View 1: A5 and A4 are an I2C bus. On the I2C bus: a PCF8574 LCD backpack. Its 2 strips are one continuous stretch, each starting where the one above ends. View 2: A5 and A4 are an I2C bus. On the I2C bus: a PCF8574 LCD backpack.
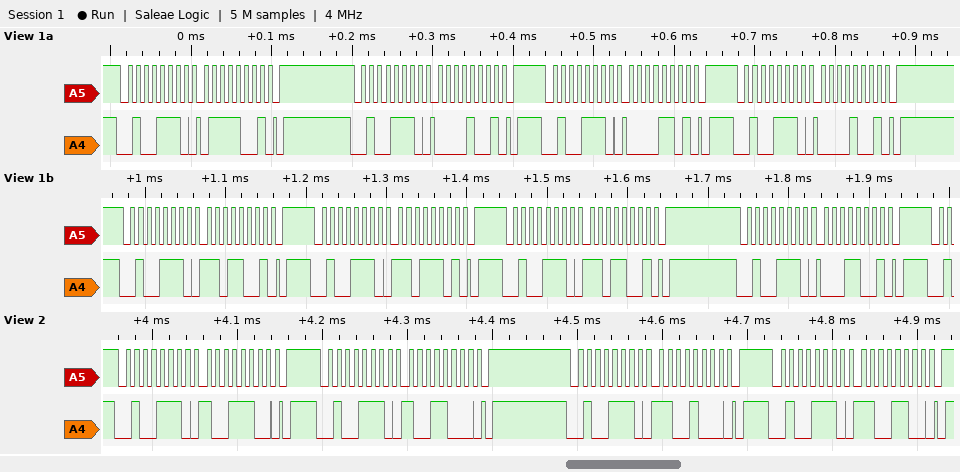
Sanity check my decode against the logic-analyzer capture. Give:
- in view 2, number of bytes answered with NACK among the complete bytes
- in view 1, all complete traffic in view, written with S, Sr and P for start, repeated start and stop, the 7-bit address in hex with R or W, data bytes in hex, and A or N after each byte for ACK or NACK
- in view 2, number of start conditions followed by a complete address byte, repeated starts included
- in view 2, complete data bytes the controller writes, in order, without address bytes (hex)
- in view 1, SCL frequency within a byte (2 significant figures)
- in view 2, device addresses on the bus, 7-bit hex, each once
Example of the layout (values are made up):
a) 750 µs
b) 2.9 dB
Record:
a) 0
b) S 27W A 79 A P S 27W A 09 A P S 27W A 0D A P S 27W A 09 A P S 27W A D9 A P S 27W A DD A P S 27W A D9 A P S 27W A 19 A P
c) 4
d) 9C 98 C8 CC
e) 100 kHz
f) 0x27
